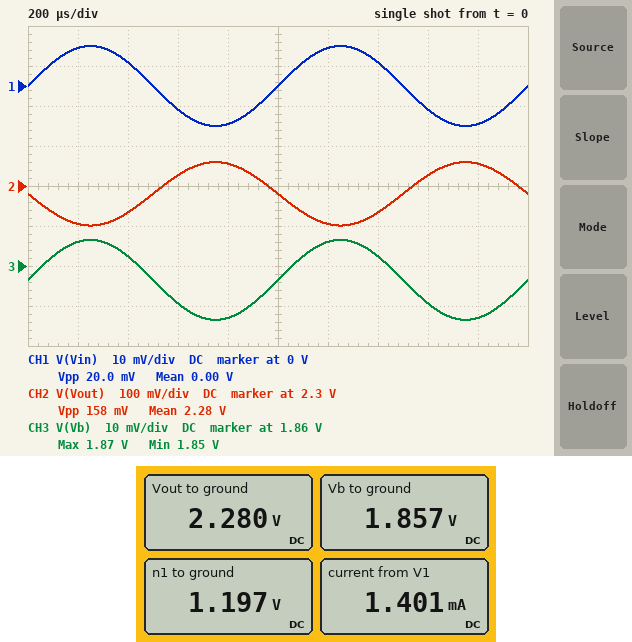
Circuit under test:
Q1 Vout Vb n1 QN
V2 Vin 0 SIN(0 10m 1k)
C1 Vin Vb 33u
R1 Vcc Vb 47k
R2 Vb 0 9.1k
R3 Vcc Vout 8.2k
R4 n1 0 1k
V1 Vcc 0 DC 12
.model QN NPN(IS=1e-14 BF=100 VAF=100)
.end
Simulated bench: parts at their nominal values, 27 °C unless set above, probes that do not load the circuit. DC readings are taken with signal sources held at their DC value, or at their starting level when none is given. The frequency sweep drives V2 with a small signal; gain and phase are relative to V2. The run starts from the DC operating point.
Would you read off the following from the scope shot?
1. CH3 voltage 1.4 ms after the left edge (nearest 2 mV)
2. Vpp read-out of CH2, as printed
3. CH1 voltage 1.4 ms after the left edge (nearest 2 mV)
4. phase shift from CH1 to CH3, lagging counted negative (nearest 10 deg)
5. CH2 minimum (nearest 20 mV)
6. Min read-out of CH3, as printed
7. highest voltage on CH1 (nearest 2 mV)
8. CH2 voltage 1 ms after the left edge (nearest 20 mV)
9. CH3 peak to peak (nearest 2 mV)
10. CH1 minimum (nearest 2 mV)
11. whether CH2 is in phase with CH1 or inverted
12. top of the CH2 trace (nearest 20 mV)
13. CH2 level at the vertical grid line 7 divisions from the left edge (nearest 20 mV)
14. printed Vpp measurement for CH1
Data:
1.862 V
158 mV
6 mV
0 deg
2.20 V
1.85 V
10 mV
2.28 V
20 mV
-10 mV
inverted
2.36 V
2.24 V
20.0 mV
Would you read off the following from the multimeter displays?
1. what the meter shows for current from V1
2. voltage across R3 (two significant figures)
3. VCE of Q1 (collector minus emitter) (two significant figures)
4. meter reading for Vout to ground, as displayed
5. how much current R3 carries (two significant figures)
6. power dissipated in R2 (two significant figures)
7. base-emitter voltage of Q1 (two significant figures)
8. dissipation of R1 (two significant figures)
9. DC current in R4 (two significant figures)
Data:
1.401 mA
9.7 V
1.1 V
2.280 V
1.2 mA
380 µW
660 mV
2.2 mW
1.2 mA
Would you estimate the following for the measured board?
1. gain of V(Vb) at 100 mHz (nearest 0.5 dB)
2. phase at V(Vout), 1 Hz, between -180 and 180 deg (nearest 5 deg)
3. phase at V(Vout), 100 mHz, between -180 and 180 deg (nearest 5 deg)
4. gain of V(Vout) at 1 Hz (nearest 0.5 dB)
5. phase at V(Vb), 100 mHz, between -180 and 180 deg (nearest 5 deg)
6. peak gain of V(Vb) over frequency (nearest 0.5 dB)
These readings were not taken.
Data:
-17.0 dB
-145 deg
-100 deg
16.5 dB
80 deg
0 dB
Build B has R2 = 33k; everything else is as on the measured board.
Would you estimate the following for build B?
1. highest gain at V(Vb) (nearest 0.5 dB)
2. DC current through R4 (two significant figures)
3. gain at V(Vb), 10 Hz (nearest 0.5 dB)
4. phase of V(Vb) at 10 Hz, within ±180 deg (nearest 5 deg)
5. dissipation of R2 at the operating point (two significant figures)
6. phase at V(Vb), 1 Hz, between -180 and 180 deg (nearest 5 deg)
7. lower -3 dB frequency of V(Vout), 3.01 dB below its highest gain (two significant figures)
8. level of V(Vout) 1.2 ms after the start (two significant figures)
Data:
0 dB
1.4 mA
-1.0 dB
30 deg
130 µW
80 deg
5.4 Hz
1.5 V
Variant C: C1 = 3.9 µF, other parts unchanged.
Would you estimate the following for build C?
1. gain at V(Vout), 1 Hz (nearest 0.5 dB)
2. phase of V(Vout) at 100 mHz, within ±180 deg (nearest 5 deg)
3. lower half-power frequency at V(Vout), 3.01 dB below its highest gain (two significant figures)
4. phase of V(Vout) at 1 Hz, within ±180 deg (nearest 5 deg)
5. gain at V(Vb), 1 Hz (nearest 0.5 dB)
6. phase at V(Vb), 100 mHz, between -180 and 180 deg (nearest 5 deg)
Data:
2.5 dB
-90 deg
5.8 Hz
-100 deg
-15.5 dB
90 deg
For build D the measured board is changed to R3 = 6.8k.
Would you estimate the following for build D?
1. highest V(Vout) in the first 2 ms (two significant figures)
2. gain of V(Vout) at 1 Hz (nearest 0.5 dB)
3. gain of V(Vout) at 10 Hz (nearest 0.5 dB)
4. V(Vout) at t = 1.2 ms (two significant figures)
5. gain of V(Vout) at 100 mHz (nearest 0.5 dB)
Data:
4.0 V
14.5 dB
16.5 dB
3.9 V
-0.5 dB
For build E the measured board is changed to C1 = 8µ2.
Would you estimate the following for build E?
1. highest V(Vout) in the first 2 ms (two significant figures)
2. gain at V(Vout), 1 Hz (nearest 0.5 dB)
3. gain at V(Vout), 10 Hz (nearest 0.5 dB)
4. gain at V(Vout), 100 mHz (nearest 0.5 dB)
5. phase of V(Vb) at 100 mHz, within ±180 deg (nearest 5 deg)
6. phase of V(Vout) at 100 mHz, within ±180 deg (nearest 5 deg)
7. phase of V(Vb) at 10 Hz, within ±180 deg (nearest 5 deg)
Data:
2.4 V
8.5 dB
17.5 dB
-11.0 dB
90 deg
-90 deg
15 deg
